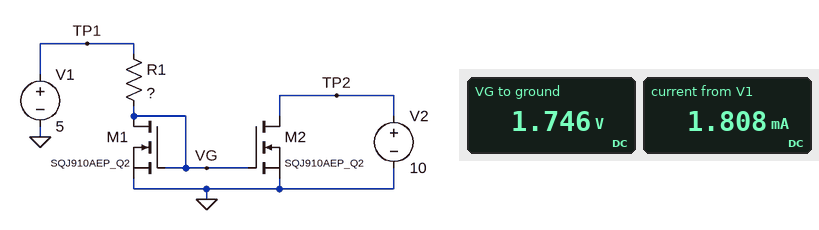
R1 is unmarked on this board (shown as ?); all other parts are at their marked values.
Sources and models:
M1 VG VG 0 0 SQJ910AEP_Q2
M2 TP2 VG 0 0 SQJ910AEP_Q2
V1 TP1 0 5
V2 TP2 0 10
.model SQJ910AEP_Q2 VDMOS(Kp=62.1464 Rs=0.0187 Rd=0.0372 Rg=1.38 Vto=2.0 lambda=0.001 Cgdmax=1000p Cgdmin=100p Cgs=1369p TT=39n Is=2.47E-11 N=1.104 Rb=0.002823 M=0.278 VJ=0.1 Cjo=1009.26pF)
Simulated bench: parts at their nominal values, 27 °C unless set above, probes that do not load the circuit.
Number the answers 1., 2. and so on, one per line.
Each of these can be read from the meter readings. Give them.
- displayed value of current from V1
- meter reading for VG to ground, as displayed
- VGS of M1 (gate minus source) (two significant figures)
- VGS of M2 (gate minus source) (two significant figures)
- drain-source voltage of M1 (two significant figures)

1. 1.808 mA
2. 1.746 V
3. 1.7 V
4. 1.7 V
5. 1.7 V
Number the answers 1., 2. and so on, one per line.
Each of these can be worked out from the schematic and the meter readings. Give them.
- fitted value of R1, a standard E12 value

1. 1.8 kΩ
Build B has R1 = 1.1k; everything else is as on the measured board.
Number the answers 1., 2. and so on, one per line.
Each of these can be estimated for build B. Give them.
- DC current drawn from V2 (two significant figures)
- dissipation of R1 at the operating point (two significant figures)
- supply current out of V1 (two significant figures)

1. 3.0 mA
2. 9.5 mW
3. 2.9 mA
